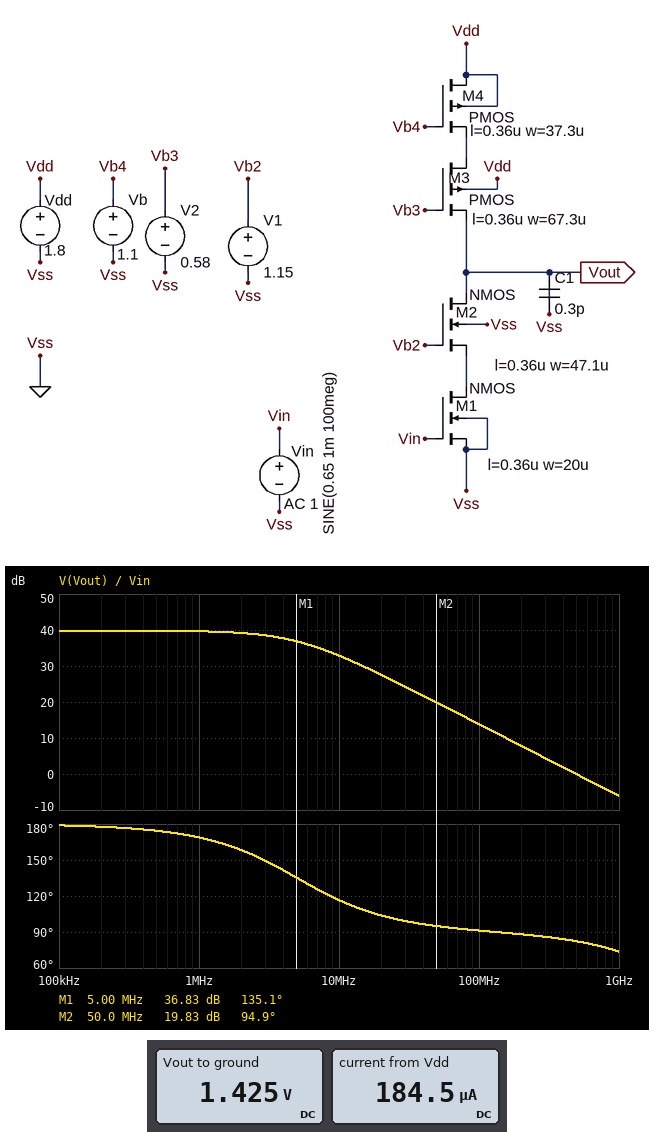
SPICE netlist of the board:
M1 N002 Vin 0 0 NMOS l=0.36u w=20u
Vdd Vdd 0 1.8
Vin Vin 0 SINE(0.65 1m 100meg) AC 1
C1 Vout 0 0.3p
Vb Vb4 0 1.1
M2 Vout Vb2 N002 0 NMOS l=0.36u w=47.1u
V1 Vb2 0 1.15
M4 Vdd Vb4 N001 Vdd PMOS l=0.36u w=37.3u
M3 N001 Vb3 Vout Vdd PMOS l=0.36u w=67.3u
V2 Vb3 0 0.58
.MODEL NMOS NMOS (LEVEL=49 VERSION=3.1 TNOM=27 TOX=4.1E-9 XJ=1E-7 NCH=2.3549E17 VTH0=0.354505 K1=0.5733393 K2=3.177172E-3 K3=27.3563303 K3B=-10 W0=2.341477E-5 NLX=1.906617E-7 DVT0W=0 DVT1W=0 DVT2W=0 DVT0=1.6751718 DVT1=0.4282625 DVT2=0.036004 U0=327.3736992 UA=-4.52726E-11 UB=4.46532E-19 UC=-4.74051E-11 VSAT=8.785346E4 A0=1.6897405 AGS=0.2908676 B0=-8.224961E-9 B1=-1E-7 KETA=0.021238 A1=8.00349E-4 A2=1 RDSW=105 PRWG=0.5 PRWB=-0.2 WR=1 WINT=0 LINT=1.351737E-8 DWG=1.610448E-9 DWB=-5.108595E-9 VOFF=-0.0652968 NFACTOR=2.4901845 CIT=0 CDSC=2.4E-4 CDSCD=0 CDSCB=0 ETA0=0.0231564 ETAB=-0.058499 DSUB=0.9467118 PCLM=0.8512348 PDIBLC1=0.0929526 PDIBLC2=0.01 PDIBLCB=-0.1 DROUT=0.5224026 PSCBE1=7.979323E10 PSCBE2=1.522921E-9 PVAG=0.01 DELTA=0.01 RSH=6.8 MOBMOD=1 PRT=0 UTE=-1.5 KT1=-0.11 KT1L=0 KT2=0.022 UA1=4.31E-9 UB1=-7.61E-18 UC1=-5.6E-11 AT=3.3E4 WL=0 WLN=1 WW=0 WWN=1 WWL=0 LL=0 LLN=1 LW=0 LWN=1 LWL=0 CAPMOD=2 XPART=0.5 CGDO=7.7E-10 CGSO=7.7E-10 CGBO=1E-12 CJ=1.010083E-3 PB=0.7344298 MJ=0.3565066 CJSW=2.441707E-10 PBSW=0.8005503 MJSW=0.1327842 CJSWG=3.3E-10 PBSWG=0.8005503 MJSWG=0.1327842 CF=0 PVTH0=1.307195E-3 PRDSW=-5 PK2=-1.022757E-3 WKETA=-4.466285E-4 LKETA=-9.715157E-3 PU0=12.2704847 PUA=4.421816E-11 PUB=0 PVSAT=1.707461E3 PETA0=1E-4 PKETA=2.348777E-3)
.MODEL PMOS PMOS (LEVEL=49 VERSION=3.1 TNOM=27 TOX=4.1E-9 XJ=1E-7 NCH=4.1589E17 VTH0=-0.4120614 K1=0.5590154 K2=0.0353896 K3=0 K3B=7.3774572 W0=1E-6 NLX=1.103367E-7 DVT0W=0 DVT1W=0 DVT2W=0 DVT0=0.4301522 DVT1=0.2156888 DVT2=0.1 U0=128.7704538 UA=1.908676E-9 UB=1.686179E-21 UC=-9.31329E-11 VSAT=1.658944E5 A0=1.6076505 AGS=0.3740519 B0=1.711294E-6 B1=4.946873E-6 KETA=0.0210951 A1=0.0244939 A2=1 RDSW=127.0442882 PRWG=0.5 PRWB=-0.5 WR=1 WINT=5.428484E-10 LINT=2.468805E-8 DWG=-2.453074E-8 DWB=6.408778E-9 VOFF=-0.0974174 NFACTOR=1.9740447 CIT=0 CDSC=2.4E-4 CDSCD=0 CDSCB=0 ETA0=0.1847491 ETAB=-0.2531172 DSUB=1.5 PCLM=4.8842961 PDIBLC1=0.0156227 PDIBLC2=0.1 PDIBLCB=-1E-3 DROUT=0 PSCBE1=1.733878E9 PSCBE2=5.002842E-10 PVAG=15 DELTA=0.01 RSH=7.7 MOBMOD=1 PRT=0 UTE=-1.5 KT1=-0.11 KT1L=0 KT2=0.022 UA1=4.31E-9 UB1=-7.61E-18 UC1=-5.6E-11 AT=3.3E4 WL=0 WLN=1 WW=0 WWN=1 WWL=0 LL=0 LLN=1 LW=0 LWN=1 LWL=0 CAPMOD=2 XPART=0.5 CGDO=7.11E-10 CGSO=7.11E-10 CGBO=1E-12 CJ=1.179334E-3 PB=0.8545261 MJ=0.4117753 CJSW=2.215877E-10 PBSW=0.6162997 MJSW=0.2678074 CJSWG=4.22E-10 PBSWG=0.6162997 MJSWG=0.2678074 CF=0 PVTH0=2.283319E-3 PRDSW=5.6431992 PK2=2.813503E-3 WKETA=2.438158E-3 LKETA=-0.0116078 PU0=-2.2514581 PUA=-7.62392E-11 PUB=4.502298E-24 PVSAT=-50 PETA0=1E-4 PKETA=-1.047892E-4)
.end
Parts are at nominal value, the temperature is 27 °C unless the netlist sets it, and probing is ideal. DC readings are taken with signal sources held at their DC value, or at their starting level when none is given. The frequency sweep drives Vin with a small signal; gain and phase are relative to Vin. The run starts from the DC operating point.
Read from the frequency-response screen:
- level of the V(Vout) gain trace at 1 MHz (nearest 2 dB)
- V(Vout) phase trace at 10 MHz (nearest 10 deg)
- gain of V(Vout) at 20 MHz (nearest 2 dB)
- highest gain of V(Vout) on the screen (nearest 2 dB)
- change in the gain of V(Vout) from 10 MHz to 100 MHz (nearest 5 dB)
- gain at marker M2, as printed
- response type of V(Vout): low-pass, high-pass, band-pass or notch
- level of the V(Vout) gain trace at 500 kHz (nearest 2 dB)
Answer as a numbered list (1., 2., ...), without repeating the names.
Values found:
1. 40 dB
2. 120 deg
3. 28 dB
4. 40 dB
5. -20 dB
6. 19.83 dB
7. low-pass
8. 40 dB
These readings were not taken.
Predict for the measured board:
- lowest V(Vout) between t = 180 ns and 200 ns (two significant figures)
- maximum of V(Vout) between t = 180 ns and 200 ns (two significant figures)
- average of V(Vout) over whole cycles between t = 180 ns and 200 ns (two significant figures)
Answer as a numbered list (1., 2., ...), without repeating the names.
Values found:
1. 1.4 V
2. 1.4 V
3. 1.4 V
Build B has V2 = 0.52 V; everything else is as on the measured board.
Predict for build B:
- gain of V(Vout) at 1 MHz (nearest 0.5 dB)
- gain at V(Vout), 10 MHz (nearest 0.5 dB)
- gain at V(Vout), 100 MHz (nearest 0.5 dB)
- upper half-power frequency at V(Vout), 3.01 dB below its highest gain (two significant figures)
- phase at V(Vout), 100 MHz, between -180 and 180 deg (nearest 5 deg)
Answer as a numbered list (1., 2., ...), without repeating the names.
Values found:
1. 39.0 dB
2. 32.5 dB
3. 13.5 dB
4. 5.3 MHz
5. 90 deg
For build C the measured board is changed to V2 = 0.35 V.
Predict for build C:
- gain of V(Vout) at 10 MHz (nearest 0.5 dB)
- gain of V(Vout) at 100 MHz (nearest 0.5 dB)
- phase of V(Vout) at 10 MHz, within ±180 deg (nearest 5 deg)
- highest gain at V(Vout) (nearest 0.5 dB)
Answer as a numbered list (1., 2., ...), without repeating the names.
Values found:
1. 32.5 dB
2. 13.5 dB
3. 120 deg
4. 38.5 dB
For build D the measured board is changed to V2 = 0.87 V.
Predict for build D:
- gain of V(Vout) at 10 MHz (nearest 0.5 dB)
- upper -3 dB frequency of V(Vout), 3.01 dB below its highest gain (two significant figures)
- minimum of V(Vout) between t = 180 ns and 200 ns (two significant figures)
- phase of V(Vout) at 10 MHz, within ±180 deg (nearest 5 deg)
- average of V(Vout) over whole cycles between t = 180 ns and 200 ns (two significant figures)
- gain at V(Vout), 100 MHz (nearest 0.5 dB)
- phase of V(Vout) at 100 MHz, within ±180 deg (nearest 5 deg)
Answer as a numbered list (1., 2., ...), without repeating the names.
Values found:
1. 32.0 dB
2. 8.9 MHz
3. 320 mV
4. 130 deg
5. 330 mV
6. 14.5 dB
7. 95 deg
